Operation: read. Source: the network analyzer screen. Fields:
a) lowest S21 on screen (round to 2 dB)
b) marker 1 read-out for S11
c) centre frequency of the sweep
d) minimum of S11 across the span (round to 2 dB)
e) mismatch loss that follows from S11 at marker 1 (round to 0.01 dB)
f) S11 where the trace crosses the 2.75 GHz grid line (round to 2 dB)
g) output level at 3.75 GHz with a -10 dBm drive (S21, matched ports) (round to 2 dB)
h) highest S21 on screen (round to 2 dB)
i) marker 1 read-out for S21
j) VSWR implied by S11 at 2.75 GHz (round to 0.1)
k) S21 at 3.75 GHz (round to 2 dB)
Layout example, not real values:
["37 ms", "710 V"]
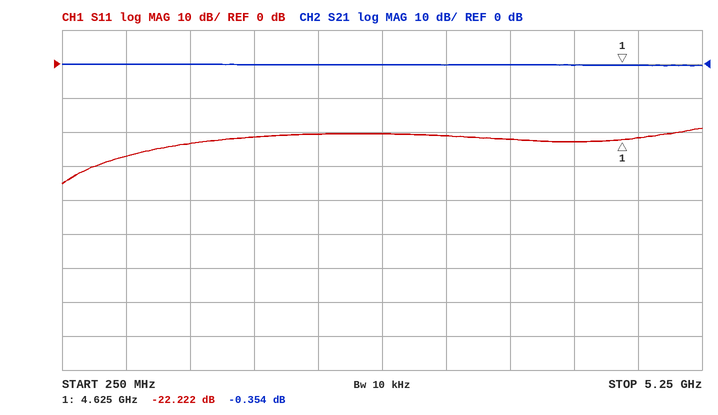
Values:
["0 dB", "-22.222 dB", "2.75 GHz", "-36 dB", "0.03 dB", "-20 dB", "-10 dBm", "0 dB", "-0.354 dB", "1.2", "0 dB"]
